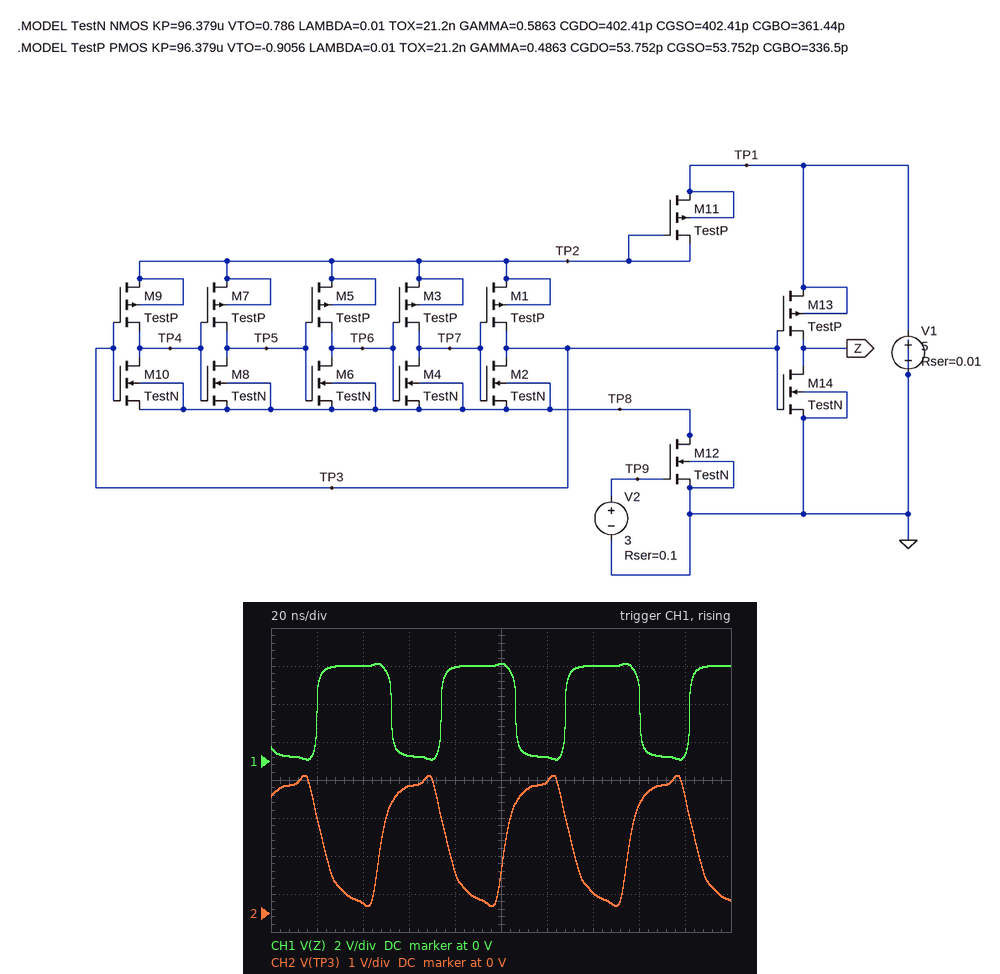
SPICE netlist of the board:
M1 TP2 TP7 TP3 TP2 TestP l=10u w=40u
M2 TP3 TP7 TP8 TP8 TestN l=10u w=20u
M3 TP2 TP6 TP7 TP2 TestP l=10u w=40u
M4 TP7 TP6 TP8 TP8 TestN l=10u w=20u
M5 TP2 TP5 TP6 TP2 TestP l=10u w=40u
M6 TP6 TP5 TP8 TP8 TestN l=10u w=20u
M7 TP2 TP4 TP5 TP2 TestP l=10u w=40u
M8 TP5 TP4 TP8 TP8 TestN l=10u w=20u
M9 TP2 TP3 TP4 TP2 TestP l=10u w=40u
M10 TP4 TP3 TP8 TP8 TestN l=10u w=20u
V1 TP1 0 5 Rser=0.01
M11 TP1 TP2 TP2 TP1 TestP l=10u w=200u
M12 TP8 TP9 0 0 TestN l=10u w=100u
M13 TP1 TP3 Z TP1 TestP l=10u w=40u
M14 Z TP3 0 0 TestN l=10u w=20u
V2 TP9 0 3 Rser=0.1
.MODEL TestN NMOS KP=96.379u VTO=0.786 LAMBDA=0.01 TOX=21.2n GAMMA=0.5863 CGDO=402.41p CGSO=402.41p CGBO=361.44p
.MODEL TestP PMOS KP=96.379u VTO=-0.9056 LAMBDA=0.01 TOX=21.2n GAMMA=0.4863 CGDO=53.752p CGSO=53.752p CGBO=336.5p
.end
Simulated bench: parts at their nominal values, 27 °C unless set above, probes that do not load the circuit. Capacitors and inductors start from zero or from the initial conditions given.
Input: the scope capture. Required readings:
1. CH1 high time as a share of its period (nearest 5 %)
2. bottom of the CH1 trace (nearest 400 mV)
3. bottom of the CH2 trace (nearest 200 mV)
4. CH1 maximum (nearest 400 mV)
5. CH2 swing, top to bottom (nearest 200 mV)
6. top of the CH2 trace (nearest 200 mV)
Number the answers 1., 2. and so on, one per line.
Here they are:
1. 60 %
2. 0 V
3. 200 mV
4. 5.2 V
5. 3.4 V
6. 3.6 V
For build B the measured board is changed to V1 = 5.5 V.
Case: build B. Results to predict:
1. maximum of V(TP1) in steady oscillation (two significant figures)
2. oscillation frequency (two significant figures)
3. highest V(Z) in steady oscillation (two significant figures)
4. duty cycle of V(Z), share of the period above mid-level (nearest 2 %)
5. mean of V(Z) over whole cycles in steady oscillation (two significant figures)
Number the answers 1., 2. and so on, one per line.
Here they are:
1. 5.5 V
2. 22 MHz
3. 5.6 V
4. 60 %
5. 3.4 V
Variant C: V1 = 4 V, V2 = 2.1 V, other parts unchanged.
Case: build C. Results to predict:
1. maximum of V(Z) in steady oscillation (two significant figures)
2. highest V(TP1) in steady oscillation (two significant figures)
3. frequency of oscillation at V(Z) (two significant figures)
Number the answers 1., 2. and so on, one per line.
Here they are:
1. 4.1 V
2. 4.0 V
3. 11 MHz
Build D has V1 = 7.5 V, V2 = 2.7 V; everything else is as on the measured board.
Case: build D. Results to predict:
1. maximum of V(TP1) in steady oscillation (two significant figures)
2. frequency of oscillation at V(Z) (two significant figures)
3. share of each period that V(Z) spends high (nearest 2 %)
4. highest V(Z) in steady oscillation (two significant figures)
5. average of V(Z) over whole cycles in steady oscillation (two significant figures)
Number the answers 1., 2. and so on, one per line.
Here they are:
1. 7.5 V
2. 34 MHz
3. 58 %
4. 7.6 V
5. 4.5 V
